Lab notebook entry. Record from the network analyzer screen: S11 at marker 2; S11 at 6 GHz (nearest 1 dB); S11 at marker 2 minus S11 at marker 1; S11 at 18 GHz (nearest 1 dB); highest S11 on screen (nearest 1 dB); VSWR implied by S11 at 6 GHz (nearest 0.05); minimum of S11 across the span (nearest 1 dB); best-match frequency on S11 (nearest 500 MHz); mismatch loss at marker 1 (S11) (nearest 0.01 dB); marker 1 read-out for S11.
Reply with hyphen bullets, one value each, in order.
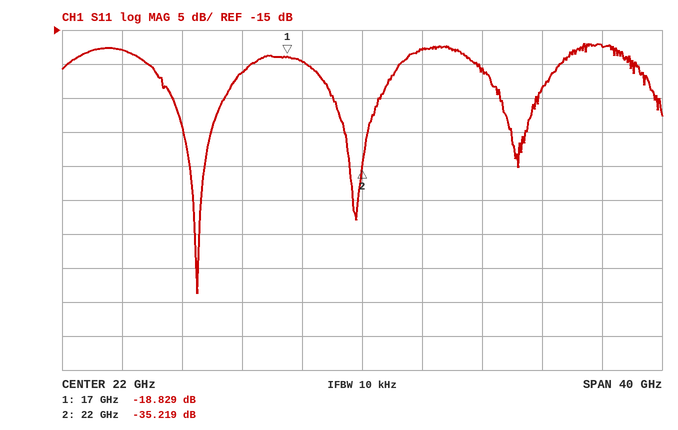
- -35.219 dB
- -18 dB
- -16.390 dB
- -20 dB
- -17 dB
- 1.30
- -54 dB
- 11.0 GHz
- 0.06 dB
- -18.829 dB
